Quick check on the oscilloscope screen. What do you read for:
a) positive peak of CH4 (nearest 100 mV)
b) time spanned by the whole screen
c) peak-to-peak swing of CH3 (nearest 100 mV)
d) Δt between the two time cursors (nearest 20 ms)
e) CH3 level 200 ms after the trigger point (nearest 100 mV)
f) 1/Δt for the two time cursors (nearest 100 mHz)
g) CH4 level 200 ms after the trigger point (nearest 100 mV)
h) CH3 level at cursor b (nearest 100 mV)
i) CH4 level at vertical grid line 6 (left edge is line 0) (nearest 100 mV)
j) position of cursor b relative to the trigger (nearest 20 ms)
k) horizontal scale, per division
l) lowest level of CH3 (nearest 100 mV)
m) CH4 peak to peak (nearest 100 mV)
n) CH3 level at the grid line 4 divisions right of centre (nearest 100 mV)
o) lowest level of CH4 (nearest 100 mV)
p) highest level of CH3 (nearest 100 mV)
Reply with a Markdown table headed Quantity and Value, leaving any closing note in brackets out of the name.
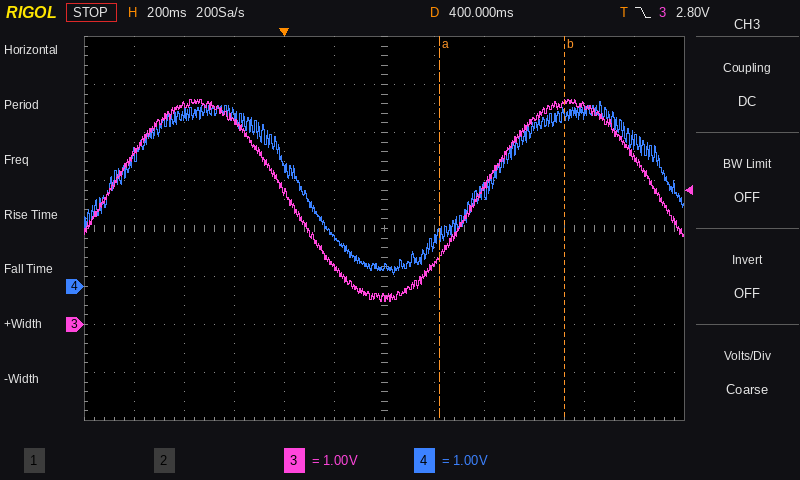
| Quantity | Value |
|---|---|
| positive peak of CH4 | 3.8 V |
| time spanned by the whole screen | 2.4 s |
| peak-to-peak swing of CH3 | 4.2 V |
| Δt between the two time cursors | 500 ms |
| CH3 level 200 ms after the trigger point | 1.2 V |
| 1/Δt for the two time cursors | 2.0 Hz |
| CH4 level 200 ms after the trigger point | 1.0 V |
| CH3 level at cursor b | 4.6 V |
| CH4 level at vertical grid line 6 (left edge is line 0) | 400 mV |
| position of cursor b relative to the trigger | +1.12 s |
| horizontal scale, per division | 200 ms |
| lowest level of CH3 | 500 mV |
| CH4 peak to peak | 3.6 V |
| CH3 level at the grid line 4 divisions right of centre | 4.6 V |
| lowest level of CH4 | 200 mV |
| highest level of CH3 | 4.7 V |
